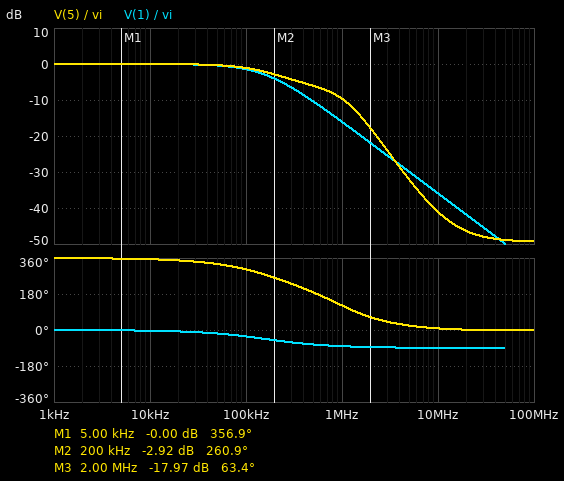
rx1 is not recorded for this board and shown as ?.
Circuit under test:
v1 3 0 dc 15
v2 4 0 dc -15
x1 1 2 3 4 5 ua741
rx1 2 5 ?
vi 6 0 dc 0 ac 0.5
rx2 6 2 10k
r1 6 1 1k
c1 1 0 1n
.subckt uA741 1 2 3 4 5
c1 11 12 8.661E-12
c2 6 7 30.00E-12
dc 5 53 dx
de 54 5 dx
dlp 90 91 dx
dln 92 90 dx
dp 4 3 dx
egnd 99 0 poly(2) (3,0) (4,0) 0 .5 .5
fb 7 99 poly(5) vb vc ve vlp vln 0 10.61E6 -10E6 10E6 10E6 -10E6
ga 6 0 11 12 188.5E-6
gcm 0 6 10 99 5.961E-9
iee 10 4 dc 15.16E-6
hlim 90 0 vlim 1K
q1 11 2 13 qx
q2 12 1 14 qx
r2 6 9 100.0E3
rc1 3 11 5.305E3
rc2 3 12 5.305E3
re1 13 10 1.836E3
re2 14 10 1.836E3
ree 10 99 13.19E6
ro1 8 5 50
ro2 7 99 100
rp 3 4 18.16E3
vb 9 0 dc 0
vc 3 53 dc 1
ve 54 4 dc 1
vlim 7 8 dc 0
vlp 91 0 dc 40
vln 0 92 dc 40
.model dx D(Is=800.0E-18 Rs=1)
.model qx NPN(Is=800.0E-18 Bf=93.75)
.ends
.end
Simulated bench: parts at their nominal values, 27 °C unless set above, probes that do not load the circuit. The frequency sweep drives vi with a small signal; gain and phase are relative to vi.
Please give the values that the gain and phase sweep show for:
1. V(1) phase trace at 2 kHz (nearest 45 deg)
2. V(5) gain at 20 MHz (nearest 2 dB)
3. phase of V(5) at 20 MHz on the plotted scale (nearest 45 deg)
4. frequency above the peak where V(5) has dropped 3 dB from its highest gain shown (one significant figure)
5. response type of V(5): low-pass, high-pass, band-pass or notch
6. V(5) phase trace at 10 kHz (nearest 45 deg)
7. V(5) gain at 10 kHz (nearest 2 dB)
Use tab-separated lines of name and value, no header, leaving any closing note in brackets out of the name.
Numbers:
V(1) phase trace at 2 kHz	0 deg
V(5) gain at 20 MHz	-46 dB
phase of V(5) at 20 MHz on the plotted scale	0 deg
frequency above the peak where V(5) has dropped 3 dB from its highest gain shown	200 kHz
response type of V(5): low-pass, high-pass, band-pass or notch	low-pass
V(5) phase trace at 10 kHz	360 deg
V(5) gain at 10 kHz	0 dB
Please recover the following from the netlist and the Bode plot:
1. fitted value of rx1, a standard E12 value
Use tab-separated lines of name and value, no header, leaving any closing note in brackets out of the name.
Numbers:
fitted value of rx1, a standard E12 value	4.7 kΩ
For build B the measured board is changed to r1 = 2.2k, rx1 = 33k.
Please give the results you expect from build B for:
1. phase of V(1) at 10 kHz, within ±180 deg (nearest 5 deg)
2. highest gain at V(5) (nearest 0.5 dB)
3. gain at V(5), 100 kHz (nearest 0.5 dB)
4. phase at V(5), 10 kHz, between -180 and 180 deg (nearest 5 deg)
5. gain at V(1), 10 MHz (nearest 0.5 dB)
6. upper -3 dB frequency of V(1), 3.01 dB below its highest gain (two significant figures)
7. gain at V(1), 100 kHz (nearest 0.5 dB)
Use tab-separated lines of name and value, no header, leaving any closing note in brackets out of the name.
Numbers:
phase of V(1) at 10 kHz, within ±180 deg	-10 deg
highest gain at V(5)	8.5 dB
gain at V(5), 100 kHz	8.0 dB
phase at V(5), 10 kHz, between -180 and 180 deg	-35 deg
gain at V(1), 10 MHz	-43.0 dB
upper -3 dB frequency of V(1), 3.01 dB below its highest gain	72 kHz
gain at V(1), 100 kHz	-4.5 dB
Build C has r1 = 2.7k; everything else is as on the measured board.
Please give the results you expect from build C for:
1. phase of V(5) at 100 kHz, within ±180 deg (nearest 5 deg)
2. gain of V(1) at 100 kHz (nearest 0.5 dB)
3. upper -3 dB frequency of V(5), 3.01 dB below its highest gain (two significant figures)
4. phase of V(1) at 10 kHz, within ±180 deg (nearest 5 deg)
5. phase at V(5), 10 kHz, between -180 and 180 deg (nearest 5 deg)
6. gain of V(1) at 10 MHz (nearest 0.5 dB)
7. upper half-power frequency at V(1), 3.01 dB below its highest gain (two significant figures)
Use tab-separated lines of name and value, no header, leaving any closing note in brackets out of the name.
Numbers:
phase of V(5) at 100 kHz, within ±180 deg	-105 deg
gain of V(1) at 100 kHz	-6.0 dB
upper -3 dB frequency of V(5), 3.01 dB below its highest gain	78 kHz
phase of V(1) at 10 kHz, within ±180 deg	-10 deg
phase at V(5), 10 kHz, between -180 and 180 deg	-15 deg
gain of V(1) at 10 MHz	-44.5 dB
upper half-power frequency at V(1), 3.01 dB below its highest gain	59 kHz
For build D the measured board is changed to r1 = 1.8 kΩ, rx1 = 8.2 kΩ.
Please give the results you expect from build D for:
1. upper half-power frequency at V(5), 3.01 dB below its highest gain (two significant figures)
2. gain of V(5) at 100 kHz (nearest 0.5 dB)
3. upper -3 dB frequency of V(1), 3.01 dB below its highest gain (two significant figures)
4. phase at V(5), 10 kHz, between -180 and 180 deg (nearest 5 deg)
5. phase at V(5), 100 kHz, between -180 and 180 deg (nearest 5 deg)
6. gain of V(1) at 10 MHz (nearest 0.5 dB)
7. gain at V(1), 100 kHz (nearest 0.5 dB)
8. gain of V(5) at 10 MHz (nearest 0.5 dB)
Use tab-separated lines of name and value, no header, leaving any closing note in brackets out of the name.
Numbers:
upper half-power frequency at V(5), 3.01 dB below its highest gain	490 kHz
gain of V(5) at 100 kHz	-1.0 dB
upper -3 dB frequency of V(1), 3.01 dB below its highest gain	88 kHz
phase at V(5), 10 kHz, between -180 and 180 deg	-15 deg
phase at V(5), 100 kHz, between -180 and 180 deg	-100 deg
gain of V(1) at 10 MHz	-41.0 dB
gain at V(1), 100 kHz	-3.5 dB
gain of V(5) at 10 MHz	-39.5 dB
